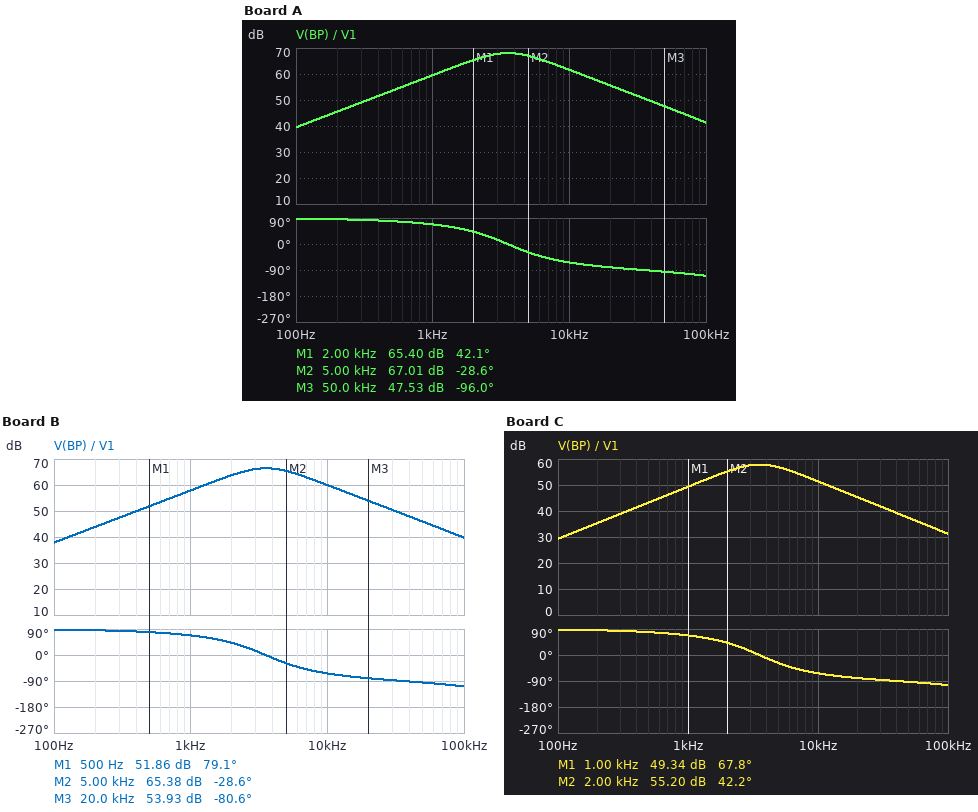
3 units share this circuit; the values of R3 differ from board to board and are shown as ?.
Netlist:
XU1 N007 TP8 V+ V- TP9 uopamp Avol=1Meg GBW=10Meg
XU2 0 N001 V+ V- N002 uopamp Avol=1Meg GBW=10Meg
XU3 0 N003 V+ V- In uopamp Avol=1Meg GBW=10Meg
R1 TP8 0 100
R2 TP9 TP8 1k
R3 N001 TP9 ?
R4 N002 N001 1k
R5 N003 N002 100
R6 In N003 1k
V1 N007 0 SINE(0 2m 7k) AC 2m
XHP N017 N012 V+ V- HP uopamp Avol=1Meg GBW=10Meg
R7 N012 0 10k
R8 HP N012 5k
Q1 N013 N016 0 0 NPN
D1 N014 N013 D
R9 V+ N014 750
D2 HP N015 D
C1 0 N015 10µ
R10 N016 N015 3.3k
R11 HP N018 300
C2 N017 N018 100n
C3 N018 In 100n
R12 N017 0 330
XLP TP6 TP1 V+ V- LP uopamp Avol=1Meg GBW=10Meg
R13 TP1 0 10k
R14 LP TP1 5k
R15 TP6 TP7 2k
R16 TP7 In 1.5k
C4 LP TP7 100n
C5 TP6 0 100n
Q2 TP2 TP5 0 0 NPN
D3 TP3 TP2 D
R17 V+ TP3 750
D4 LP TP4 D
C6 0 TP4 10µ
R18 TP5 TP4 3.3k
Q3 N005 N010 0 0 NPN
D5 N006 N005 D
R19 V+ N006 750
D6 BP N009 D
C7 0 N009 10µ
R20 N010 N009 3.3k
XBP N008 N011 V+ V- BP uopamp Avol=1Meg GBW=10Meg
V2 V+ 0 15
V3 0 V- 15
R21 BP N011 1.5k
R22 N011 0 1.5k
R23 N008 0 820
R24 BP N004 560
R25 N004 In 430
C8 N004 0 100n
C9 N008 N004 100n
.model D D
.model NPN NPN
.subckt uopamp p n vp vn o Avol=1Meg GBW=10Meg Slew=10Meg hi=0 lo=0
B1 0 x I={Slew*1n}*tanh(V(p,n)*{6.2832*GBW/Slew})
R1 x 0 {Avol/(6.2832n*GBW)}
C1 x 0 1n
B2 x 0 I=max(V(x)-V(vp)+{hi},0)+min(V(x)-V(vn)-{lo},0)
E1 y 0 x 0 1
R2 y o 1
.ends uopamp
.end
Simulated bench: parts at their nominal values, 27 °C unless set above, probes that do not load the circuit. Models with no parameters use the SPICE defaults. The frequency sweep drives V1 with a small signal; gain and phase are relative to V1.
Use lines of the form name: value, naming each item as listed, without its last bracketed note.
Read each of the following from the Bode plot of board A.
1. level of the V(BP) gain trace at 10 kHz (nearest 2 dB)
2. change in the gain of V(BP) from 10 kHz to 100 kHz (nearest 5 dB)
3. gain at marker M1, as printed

level of the V(BP) gain trace at 10 kHz: 62 dB
change in the gain of V(BP) from 10 kHz to 100 kHz: -20 dB
gain at marker M1, as printed: 65.40 dB
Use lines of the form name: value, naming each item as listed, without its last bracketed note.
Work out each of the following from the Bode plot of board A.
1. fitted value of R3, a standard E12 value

fitted value of R3, a standard E12 value: 68 Ω
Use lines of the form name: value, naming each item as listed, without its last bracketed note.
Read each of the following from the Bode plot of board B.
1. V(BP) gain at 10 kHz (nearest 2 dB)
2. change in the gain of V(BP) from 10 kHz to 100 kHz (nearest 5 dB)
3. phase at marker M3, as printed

V(BP) gain at 10 kHz: 60 dB
change in the gain of V(BP) from 10 kHz to 100 kHz: -20 dB
phase at marker M3, as printed: -80.6 deg
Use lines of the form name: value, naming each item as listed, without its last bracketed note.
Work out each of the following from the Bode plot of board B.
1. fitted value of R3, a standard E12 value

fitted value of R3, a standard E12 value: 82 Ω
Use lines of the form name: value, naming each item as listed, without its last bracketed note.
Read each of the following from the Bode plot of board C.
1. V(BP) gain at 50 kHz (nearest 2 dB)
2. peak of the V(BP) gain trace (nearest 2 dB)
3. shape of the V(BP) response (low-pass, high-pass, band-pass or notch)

V(BP) gain at 50 kHz: 38 dB
peak of the V(BP) gain trace: 58 dB
shape of the V(BP) response: band-pass
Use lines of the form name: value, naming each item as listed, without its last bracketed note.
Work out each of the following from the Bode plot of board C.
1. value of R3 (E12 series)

value of R3: 220 Ω
